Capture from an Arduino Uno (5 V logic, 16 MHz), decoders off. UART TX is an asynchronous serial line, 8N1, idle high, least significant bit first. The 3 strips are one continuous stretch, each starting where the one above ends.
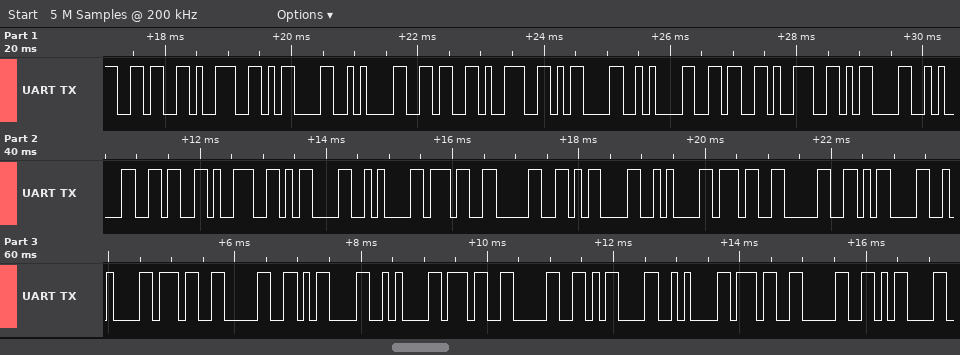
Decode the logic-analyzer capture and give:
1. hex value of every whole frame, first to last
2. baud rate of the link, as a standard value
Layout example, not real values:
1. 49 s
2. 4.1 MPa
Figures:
1. 36 39 0D 0A 36 39 0D 0A 36 39 0D 0A 36 39 0D 0A 37 30 0D 0A 37 30 0D 0A 37 30 0D 0A 37 30 0D 0A 37 30 0D
2. 9600 baud
